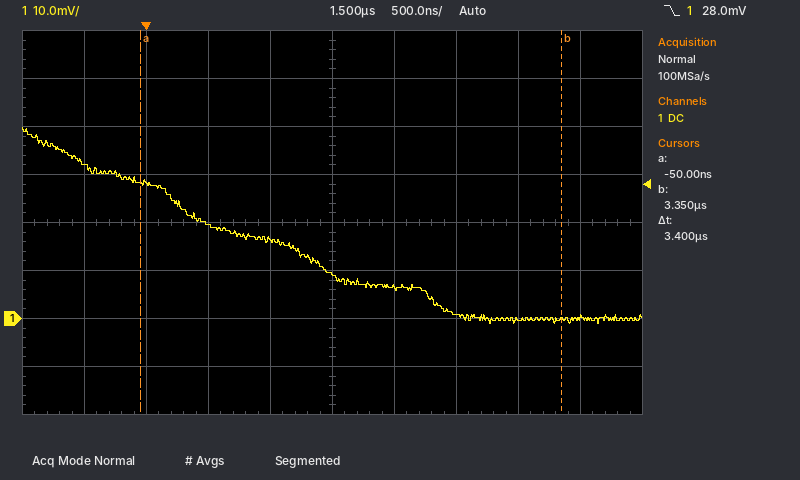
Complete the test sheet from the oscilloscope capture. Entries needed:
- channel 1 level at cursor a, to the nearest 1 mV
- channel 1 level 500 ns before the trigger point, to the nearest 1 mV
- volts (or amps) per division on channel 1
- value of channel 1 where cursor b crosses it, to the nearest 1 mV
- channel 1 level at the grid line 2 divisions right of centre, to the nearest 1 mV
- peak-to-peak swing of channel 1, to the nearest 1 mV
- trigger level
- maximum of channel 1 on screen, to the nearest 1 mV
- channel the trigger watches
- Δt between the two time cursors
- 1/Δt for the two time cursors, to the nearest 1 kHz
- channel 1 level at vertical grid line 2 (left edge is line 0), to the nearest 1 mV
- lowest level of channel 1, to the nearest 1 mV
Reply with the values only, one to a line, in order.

28 mV
32 mV
10 mV
0 mV
1 mV
41 mV
28.0 mV
40 mV
channel 1
3.4 µs
294 kHz
28 mV
-1 mV
